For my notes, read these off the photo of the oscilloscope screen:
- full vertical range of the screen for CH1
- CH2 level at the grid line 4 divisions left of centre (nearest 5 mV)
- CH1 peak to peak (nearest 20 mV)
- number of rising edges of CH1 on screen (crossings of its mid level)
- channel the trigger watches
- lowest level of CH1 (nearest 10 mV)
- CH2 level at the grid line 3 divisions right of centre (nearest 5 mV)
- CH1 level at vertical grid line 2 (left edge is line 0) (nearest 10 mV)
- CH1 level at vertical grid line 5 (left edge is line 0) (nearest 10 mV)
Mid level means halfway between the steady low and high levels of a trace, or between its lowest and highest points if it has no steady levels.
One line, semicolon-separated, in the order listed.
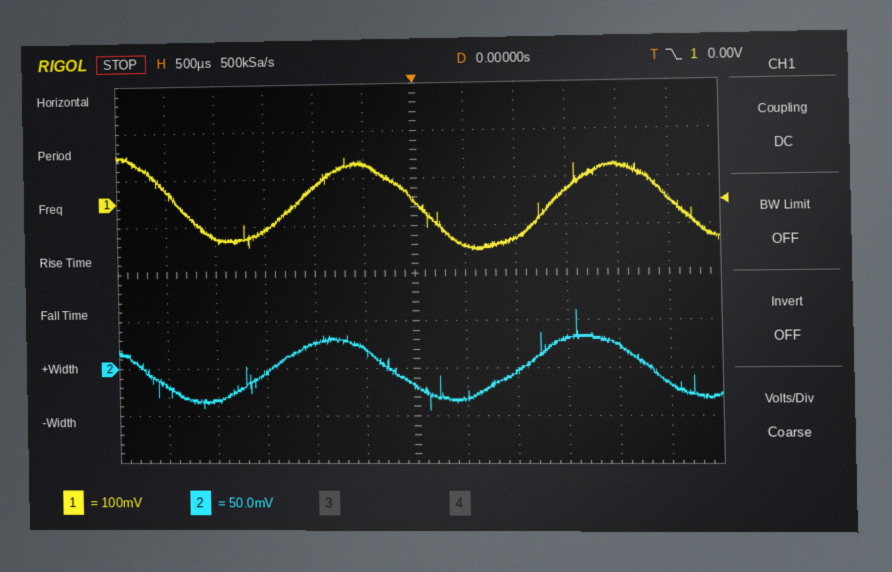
800 mV; -35 mV; 200 mV; 2; CH1; -100 mV; 30 mV; -70 mV; 80 mV
